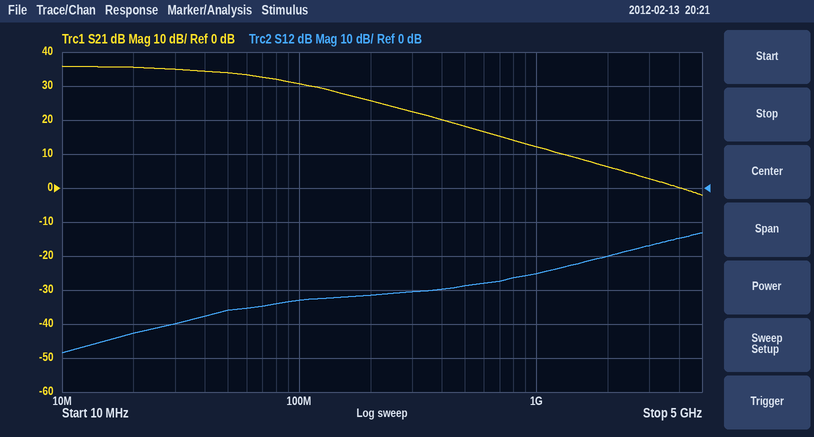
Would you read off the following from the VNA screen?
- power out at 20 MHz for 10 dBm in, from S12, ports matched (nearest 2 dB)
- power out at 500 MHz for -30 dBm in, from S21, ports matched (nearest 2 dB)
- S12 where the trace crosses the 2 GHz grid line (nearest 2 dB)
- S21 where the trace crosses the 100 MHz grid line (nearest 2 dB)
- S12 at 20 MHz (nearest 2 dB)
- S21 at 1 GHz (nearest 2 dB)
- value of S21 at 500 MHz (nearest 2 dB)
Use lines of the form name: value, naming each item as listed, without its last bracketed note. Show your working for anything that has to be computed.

power out at 20 MHz for 10 dBm in, from S12, ports matched: 10 dBm + (-42 dB) = -32 dBm
power out at 500 MHz for -30 dBm in, from S21, ports matched: -30 dBm + (18 dB) = -12 dBm
S12 where the trace crosses the 2 GHz grid line: -20 dB
S21 where the trace crosses the 100 MHz grid line: 30 dB
S12 at 20 MHz: -42 dB
S21 at 1 GHz: 12 dB
value of S21 at 500 MHz: 18 dB
